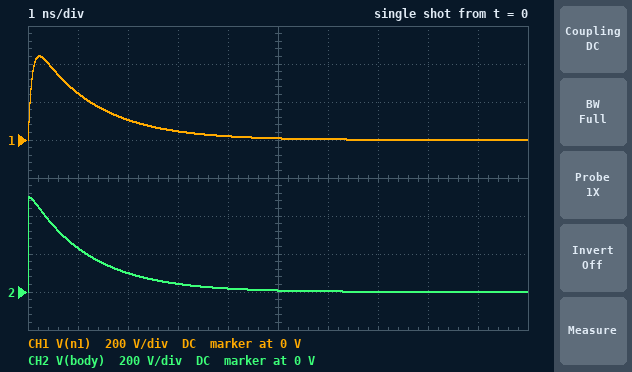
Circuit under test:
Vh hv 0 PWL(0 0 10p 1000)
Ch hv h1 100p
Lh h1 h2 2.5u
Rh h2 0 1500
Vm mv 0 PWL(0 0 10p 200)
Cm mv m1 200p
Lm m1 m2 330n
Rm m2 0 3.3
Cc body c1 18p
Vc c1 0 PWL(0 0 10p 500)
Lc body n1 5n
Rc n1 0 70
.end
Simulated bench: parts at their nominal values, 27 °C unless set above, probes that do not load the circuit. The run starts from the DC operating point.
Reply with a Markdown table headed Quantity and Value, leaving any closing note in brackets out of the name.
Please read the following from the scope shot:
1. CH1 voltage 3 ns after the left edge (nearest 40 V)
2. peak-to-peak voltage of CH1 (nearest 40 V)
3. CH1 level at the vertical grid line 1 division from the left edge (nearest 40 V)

| Quantity | Value |
|---|---|
| CH1 voltage 3 ns after the left edge | 40 V |
| peak-to-peak voltage of CH1 | 440 V |
| CH1 level at the vertical grid line 1 division from the left edge | 240 V |
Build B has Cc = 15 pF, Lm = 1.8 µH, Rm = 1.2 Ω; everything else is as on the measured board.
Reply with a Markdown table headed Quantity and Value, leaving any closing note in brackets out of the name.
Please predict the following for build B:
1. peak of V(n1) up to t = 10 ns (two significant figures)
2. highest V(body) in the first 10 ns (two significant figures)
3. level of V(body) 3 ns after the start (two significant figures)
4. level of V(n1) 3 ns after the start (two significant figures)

| Quantity | Value |
|---|---|
| peak of V(n1) up to t = 10 ns | 430 V |
| highest V(body) in the first 10 ns | 500 V |
| level of V(body) 3 ns after the start | 25 V |
| level of V(n1) 3 ns after the start | 27 V |
